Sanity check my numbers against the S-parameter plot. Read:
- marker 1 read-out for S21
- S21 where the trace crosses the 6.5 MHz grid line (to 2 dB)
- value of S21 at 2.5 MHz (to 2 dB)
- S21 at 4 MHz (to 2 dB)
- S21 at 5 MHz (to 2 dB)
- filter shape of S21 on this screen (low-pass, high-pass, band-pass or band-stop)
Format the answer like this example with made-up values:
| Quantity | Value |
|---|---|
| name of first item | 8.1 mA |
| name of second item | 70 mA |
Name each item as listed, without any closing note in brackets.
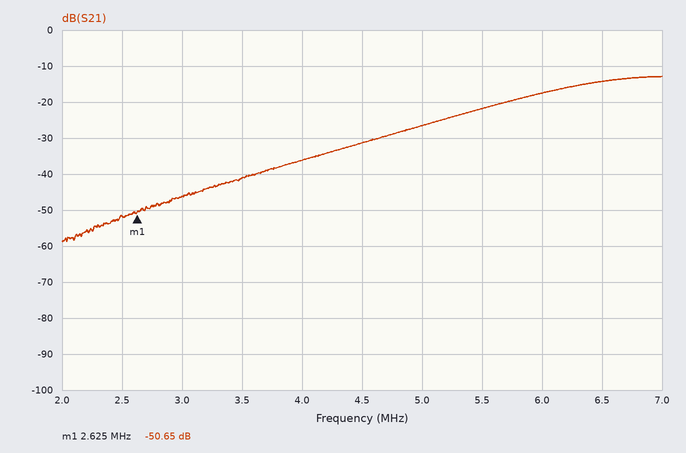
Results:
| Quantity | Value |
|---|---|
| marker 1 read-out for S21 | -50.65 dB |
| S21 where the trace crosses the 6.5 MHz grid line | -14 dB |
| value of S21 at 2.5 MHz | -52 dB |
| S21 at 4 MHz | -36 dB |
| S21 at 5 MHz | -26 dB |
| filter shape of S21 on this screen | high-pass |
